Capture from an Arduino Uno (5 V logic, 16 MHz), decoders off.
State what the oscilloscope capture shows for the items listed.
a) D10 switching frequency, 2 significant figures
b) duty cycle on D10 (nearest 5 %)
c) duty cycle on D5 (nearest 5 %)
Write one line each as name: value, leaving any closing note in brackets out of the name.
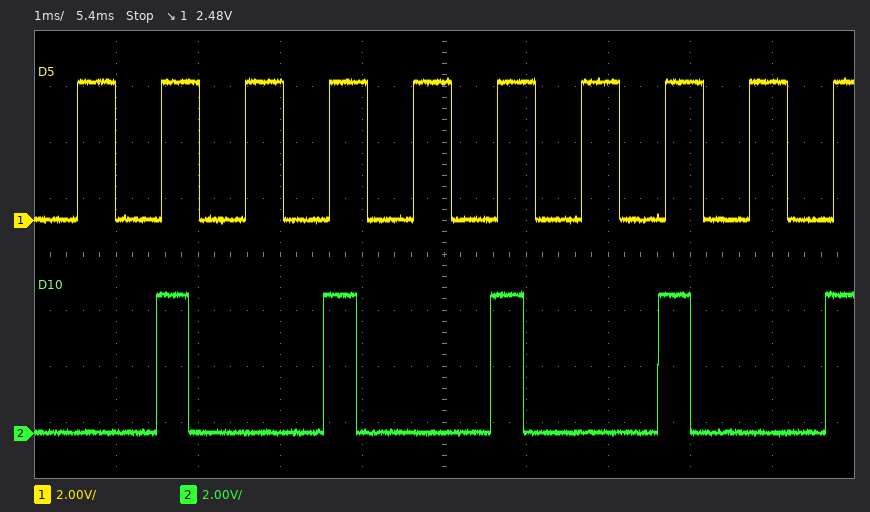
D10 switching frequency, 2 significant figures: 490 Hz
duty cycle on D10: 20 %
duty cycle on D5: 45 %
